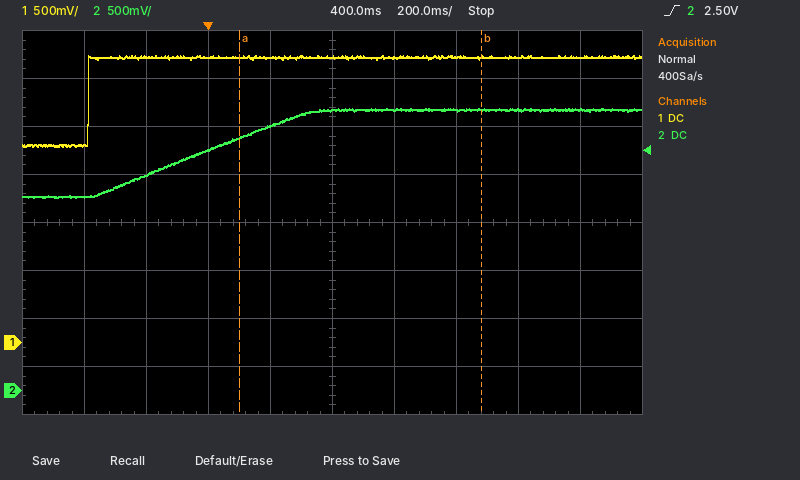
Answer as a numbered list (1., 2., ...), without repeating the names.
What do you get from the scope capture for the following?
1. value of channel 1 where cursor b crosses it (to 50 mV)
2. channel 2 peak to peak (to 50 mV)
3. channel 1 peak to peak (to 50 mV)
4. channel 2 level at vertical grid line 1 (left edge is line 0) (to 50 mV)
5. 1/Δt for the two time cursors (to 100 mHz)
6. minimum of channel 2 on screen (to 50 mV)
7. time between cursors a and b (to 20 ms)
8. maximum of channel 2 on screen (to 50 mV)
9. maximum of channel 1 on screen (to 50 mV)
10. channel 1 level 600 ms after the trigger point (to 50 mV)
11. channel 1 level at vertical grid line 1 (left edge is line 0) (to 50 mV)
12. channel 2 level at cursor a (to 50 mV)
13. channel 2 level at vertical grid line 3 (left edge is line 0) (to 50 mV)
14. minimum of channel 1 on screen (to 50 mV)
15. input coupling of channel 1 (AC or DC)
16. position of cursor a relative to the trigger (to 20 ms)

1. 2.95 V
2. 950 mV
3. 950 mV
4. 2.00 V
5. 1.3 Hz
6. 2.00 V
7. 780 ms
8. 2.95 V
9. 3.00 V
10. 2.95 V
11. 2.05 V
12. 2.65 V
13. 2.50 V
14. 2.05 V
15. DC
16. +100 ms
